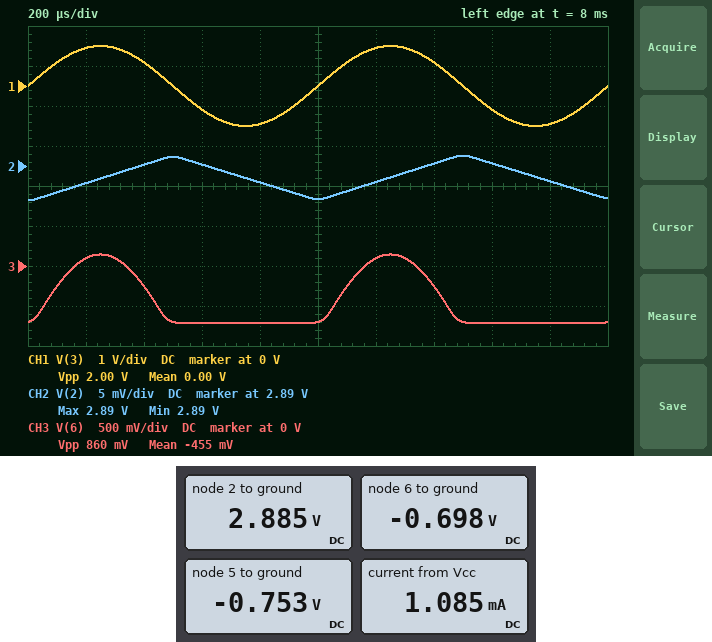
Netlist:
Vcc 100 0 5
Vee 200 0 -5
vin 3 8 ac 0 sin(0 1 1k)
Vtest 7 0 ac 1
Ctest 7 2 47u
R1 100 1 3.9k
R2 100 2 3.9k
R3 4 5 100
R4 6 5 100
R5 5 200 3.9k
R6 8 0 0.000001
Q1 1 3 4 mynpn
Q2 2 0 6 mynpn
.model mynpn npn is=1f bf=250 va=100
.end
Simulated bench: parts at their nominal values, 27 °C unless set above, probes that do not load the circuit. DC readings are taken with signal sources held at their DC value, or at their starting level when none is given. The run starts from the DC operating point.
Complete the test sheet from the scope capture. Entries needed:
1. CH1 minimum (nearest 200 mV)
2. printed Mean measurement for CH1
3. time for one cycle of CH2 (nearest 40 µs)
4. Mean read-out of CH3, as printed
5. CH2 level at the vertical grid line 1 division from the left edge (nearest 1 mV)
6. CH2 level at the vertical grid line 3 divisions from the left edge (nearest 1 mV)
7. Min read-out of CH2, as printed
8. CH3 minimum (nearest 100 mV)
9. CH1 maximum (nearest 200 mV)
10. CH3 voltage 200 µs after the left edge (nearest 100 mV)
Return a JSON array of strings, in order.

["-1.0 V", "0.00 V", "1.00 ms", "-455 mV", "2.888 V", "2.890 V", "2.89 V", "-700 mV", "1.0 V", "100 mV"]
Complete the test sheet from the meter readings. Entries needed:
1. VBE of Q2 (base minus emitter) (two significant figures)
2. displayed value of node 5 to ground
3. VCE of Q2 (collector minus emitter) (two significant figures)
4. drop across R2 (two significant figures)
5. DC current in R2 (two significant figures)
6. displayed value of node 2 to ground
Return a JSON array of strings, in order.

["700 mV", "-0.753 V", "3.6 V", "2.1 V", "540 µA", "2.885 V"]
